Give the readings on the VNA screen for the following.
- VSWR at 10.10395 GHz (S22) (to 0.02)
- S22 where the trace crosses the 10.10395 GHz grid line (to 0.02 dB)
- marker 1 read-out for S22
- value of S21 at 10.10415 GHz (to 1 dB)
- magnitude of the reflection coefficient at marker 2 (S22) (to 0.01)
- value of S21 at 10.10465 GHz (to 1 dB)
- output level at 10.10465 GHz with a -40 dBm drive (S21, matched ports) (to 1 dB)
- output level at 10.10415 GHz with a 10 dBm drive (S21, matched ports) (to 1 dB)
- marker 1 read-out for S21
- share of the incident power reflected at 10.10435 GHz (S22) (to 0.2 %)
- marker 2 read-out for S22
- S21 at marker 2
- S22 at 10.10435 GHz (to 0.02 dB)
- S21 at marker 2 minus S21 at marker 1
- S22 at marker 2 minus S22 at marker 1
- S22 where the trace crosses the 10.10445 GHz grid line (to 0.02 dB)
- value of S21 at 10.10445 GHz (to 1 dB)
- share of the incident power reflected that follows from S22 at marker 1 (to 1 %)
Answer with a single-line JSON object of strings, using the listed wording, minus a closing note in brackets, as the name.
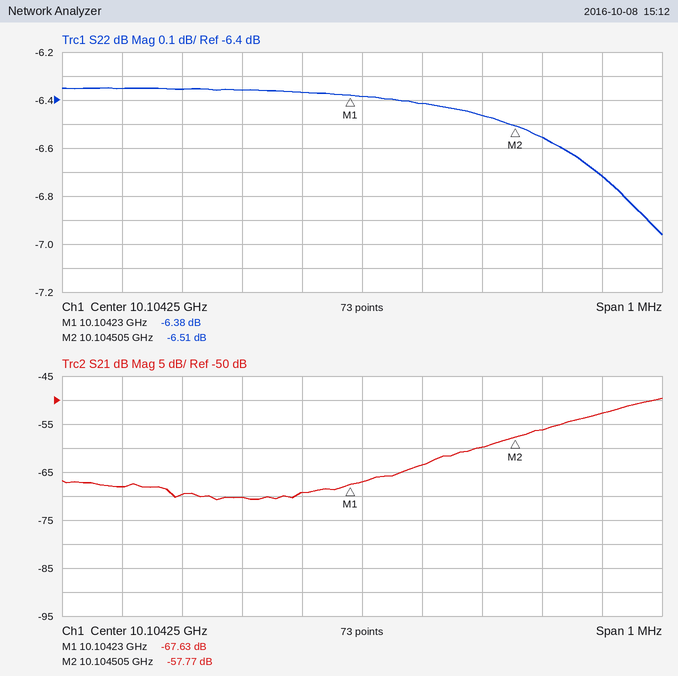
{"VSWR at 10.10395 GHz (S22)": "2.86", "S22 where the trace crosses the 10.10395 GHz grid line": "-6.36 dB", "marker 1 read-out for S22": "-6.38 dB", "value of S21 at 10.10415 GHz": "-69 dB", "magnitude of the reflection coefficient at marker 2 (S22)": "0.47", "value of S21 at 10.10465 GHz": "-53 dB", "output level at 10.10465 GHz with a -40 dBm drive (S21, matched ports)": "-93 dBm", "output level at 10.10415 GHz with a 10 dBm drive (S21, matched ports)": "-59 dBm", "marker 1 read-out for S21": "-67.63 dB", "share of the incident power reflected at 10.10435 GHz (S22)": "22.8 %", "marker 2 read-out for S22": "-6.51 dB", "S21 at marker 2": "-57.77 dB", "S22 at 10.10435 GHz": "-6.42 dB", "S21 at marker 2 minus S21 at marker 1": "9.86 dB", "S22 at marker 2 minus S22 at marker 1": "-0.13 dB", "S22 where the trace crosses the 10.10445 GHz grid line": "-6.46 dB", "value of S21 at 10.10445 GHz": "-60 dB", "share of the incident power reflected that follows from S22 at marker 1": "23 %"}
